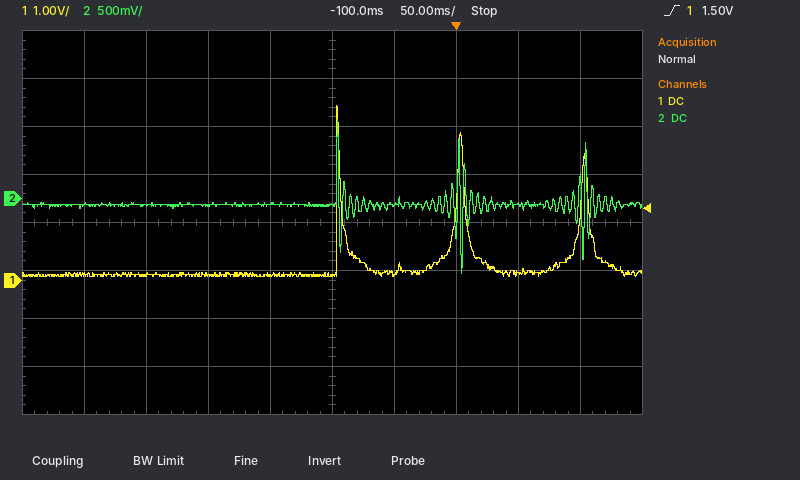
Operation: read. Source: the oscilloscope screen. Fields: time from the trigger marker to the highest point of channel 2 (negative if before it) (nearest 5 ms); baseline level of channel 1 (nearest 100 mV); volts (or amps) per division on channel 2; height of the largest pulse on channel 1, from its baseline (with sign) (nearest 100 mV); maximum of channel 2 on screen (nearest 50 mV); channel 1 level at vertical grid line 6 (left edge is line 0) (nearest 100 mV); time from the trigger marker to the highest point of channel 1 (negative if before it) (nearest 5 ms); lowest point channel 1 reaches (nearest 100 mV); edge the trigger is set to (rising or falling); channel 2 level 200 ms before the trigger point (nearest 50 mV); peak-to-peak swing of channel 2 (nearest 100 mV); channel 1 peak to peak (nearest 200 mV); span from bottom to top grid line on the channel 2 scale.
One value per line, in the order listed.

-95 ms
100 mV
500 mV
+3.5 V
800 mV
100 mV
-95 ms
100 mV
rising
-50 mV
1.60 V
3.6 V
4 V
